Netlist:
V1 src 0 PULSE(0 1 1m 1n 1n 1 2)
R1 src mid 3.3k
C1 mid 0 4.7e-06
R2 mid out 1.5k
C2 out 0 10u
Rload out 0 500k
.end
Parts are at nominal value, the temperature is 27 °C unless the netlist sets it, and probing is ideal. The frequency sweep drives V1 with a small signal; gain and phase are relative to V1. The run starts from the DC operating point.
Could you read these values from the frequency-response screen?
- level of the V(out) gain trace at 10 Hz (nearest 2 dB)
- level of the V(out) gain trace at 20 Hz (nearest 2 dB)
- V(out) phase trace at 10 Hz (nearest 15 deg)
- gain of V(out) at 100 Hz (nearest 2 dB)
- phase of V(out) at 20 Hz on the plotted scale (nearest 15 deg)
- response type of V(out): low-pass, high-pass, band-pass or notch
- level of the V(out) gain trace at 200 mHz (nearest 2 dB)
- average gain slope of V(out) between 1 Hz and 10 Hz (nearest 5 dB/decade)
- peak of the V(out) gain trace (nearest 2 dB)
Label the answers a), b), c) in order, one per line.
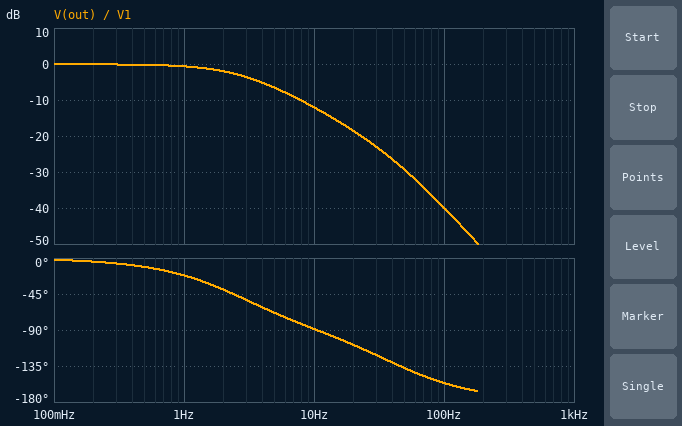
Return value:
a) -12 dB
b) -18 dB
c) -90 deg
d) -40 dB
e) -105 deg
f) low-pass
g) 0 dB
h) -10 dB/decade
i) 0 dB
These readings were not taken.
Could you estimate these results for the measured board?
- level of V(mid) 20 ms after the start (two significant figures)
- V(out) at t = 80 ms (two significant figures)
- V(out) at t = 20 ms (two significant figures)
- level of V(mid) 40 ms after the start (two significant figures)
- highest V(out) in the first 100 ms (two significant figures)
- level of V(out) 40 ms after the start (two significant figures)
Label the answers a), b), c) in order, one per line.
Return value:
a) 420 mV
b) 710 mV
c) 220 mV
d) 580 mV
e) 790 mV
f) 440 mV
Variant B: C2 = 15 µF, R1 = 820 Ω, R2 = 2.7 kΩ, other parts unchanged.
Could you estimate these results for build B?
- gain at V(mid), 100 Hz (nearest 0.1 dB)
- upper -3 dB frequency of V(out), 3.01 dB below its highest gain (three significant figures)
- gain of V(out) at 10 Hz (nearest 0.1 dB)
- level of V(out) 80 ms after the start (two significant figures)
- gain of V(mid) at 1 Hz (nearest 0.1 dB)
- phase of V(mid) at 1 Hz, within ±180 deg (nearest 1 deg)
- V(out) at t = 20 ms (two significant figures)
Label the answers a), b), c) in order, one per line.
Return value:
a) -8.8 dB
b) 2.97 Hz
c) -11.1 dB
d) 750 mV
e) -0.2 dB
f) -5 deg
g) 260 mV
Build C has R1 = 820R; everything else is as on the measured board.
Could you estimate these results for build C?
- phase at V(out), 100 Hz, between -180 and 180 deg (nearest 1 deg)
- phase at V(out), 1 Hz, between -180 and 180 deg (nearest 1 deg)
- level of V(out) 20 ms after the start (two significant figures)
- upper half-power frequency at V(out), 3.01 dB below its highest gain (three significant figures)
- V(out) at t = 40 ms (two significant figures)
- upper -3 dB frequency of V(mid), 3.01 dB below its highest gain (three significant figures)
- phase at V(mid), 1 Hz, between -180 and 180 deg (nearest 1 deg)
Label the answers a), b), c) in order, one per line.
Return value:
a) -142 deg
b) -10 deg
c) 490 mV
d) 6.41 Hz
e) 770 mV
f) 11.8 Hz
g) -4 deg
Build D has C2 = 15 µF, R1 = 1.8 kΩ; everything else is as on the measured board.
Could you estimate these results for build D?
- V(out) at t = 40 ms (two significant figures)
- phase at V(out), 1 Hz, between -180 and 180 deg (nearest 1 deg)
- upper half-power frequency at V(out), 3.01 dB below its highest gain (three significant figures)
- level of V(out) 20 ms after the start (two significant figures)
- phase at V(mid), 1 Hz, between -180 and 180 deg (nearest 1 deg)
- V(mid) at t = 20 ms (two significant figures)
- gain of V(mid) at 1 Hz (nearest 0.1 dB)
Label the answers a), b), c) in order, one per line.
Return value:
a) 480 mV
b) -20 deg
c) 2.93 Hz
d) 250 mV
e) -12 deg
f) 560 mV
g) -0.4 dB
